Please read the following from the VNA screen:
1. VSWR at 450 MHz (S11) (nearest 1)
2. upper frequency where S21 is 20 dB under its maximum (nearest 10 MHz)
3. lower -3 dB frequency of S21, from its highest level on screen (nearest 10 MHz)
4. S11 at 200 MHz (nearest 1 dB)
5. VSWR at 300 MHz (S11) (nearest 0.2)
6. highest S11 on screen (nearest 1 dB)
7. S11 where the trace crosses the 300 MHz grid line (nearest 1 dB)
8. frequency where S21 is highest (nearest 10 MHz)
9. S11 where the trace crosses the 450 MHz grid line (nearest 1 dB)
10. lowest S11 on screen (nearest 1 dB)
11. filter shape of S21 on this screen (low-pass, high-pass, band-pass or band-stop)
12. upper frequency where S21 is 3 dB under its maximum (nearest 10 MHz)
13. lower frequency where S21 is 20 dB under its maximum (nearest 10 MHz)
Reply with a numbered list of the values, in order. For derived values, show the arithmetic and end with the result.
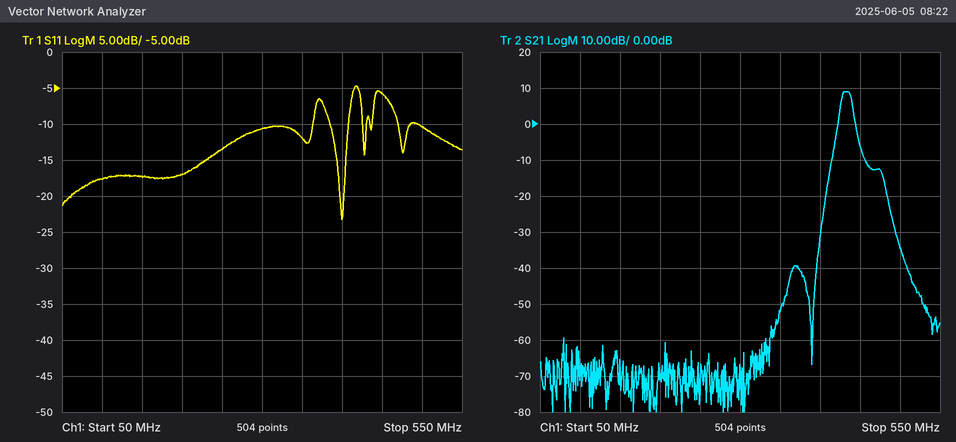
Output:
1. |Γ| = 10^(-6/20) = 0.5012; VSWR = (1 + 0.5012)/(1 − 0.5012) ≈ 3
2. 460 MHz
3. 430 MHz
4. -17 dB
5. |Γ| = 10^(-11/20) = 0.2818; VSWR = (1 + 0.2818)/(1 − 0.2818) ≈ 1.8
6. -5 dB
7. -11 dB
8. 430 MHz
9. -6 dB
10. -23 dB
11. band-pass
12. 440 MHz
13. 410 MHz
